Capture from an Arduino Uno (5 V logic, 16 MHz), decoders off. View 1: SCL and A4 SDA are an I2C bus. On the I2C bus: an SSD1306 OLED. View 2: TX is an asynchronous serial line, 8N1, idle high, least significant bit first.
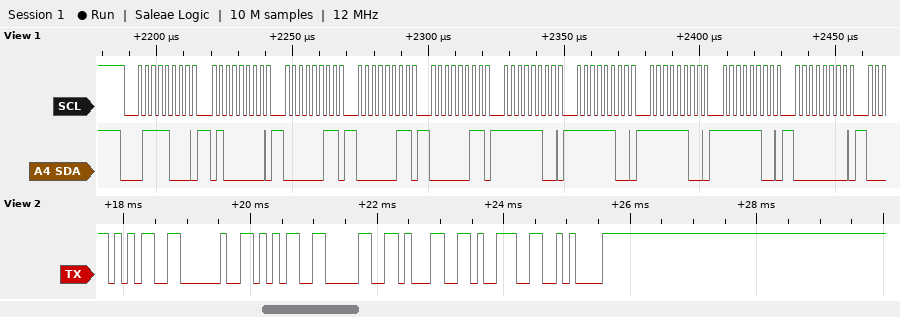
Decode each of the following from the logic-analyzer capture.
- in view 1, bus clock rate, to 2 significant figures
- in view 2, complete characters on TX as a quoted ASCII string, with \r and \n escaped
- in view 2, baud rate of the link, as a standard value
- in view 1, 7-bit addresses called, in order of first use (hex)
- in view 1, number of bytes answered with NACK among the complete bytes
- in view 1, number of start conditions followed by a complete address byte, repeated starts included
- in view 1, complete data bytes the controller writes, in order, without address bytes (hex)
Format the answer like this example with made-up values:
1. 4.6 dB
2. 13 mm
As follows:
1. 400 kHz
2. "5 5019\n"
3. 9600 baud
4. 0x3C
5. 0
6. 1
7. 40 03 03 03 FC FC FC FC 00
